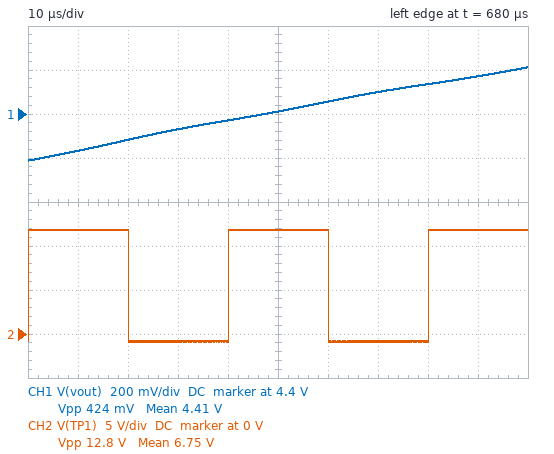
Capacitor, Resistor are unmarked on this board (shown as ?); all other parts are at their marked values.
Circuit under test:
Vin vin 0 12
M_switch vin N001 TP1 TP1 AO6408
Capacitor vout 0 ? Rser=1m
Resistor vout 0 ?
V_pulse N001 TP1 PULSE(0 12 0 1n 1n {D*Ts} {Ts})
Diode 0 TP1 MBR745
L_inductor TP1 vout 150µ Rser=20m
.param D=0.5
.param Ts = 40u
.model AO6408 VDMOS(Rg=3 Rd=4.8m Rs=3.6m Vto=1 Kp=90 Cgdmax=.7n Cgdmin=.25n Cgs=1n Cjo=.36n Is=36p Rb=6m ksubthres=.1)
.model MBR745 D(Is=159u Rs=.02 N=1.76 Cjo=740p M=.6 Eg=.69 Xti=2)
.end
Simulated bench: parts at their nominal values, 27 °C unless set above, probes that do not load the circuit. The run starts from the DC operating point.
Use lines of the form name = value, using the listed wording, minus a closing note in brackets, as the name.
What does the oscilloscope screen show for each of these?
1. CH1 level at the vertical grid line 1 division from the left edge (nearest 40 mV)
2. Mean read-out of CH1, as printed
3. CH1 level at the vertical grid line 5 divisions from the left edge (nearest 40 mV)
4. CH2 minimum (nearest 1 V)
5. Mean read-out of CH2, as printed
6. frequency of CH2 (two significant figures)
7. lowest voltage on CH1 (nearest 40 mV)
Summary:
CH1 level at the vertical grid line 1 division from the left edge = 4.24 V
Mean read-out of CH1, as printed = 4.41 V
CH1 level at the vertical grid line 5 divisions from the left edge = 4.40 V
CH2 minimum = -1 V
Mean read-out of CH2, as printed = 6.75 V
frequency of CH2 = 25 kHz
lowest voltage on CH1 = 4.20 V
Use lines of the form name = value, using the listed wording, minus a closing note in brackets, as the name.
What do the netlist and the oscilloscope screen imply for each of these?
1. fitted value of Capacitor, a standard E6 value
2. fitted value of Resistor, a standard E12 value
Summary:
fitted value of Capacitor, a standard E6 value = 680 µF
fitted value of Resistor, a standard E12 value = 0.33 Ω
